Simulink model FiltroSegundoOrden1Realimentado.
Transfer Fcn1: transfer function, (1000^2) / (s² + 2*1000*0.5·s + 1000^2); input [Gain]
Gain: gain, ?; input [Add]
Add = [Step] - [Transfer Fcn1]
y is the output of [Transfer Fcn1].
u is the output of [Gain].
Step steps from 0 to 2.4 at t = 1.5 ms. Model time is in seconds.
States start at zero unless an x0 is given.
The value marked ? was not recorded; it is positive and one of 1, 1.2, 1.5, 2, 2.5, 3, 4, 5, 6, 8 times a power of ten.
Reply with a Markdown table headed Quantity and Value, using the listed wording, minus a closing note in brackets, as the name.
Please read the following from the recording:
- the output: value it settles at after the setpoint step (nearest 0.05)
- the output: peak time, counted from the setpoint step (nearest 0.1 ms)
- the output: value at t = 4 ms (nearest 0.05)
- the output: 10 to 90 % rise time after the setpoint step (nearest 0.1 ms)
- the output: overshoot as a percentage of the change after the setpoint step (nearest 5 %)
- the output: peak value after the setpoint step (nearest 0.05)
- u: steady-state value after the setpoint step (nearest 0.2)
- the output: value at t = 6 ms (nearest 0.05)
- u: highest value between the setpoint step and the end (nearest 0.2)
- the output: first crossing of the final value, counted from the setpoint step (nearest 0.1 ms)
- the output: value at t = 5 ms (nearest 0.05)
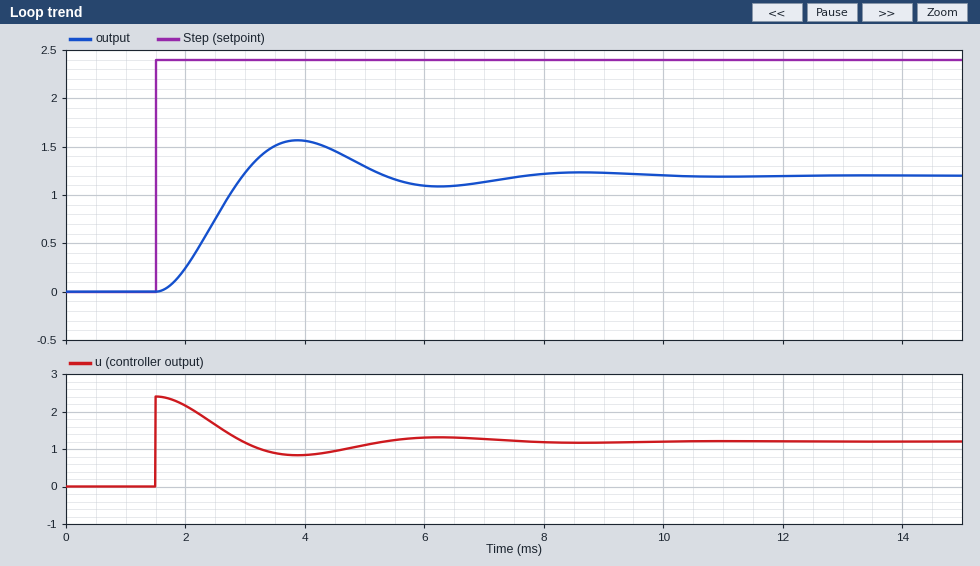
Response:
| Quantity | Value |
|---|---|
| the output: value it settles at after the setpoint step | 1.20 |
| the output: peak time, counted from the setpoint step | 2.4 ms |
| the output: value at t = 4 ms | 1.55 |
| the output: 10 to 90 % rise time after the setpoint step | 1.0 ms |
| the output: overshoot as a percentage of the change after the setpoint step | 30 % |
| the output: peak value after the setpoint step | 1.55 |
| u: steady-state value after the setpoint step | 1.2 |
| the output: value at t = 6 ms | 1.10 |
| u: highest value between the setpoint step and the end | 2.4 |
| the output: first crossing of the final value, counted from the setpoint step | 1.5 ms |
| the output: value at t = 5 ms | 1.30 |
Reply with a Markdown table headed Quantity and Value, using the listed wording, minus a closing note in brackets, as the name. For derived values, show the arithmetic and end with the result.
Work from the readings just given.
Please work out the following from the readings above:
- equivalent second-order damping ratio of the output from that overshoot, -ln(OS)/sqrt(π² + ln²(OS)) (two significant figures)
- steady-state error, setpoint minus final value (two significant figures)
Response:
| Quantity | Value |
|---|---|
| equivalent second-order damping ratio of the output from that overshoot, -ln(OS)/sqrt(π² + ln²(OS)) | ln(0.3) = -1.204; 1.204 / sqrt(9.870 + 1.450) = 0.36 |
| steady-state error, setpoint minus final value | 2.4 - 1.2 = 1.2 |
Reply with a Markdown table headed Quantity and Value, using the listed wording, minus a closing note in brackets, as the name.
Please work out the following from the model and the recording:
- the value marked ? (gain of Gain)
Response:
| Quantity | Value |
|---|---|
| the value marked ? | 1 |
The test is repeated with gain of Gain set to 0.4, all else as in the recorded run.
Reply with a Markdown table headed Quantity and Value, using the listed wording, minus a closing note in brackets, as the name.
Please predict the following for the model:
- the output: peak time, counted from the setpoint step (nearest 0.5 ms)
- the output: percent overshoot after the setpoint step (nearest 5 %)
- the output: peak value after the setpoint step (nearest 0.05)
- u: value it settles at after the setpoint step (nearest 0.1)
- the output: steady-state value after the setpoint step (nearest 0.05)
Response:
| Quantity | Value |
|---|---|
| the output: peak time, counted from the setpoint step | 3.0 ms |
| the output: percent overshoot after the setpoint step | 25 % |
| the output: peak value after the setpoint step | 0.85 |
| u: value it settles at after the setpoint step | 0.7 |
| the output: steady-state value after the setpoint step | 0.70 |
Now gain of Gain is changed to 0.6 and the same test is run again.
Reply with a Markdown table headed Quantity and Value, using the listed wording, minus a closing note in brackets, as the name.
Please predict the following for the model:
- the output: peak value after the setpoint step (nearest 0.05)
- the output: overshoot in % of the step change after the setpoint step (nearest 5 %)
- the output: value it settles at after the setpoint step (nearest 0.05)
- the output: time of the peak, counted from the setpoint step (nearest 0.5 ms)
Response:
| Quantity | Value |
|---|---|
| the output: peak value after the setpoint step | 1.15 |
| the output: overshoot in % of the step change after the setpoint step | 25 % |
| the output: value it settles at after the setpoint step | 0.90 |
| the output: time of the peak, counted from the setpoint step | 2.5 ms |
